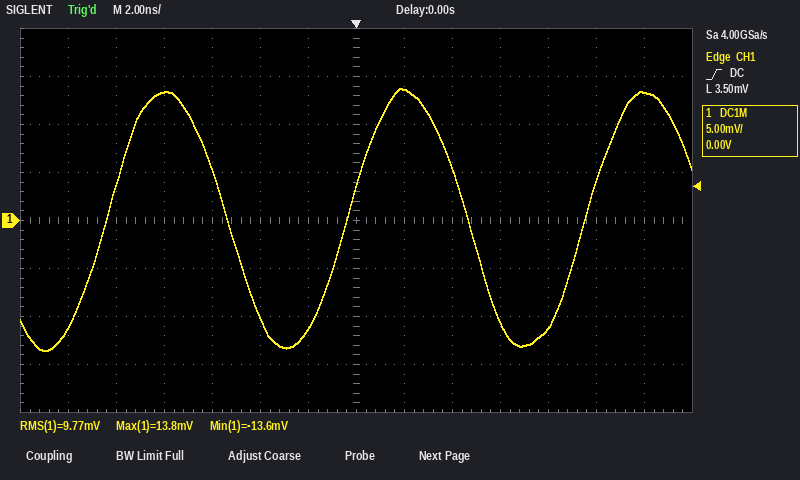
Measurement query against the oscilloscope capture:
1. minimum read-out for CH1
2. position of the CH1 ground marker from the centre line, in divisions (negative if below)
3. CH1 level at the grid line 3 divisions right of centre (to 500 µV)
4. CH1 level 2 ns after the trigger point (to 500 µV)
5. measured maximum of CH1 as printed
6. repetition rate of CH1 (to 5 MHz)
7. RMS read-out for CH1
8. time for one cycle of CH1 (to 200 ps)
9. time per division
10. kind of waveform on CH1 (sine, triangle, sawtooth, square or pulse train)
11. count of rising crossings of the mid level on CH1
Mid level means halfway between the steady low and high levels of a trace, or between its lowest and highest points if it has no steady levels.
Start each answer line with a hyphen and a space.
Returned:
- -13.6 mV
- 0.0 div
- -10.5 mV
- 13.5 mV
- 13.8 mV
- 100 MHz
- 9.77 mV
- 10.0 ns
- 2 ns
- sine
- 3
